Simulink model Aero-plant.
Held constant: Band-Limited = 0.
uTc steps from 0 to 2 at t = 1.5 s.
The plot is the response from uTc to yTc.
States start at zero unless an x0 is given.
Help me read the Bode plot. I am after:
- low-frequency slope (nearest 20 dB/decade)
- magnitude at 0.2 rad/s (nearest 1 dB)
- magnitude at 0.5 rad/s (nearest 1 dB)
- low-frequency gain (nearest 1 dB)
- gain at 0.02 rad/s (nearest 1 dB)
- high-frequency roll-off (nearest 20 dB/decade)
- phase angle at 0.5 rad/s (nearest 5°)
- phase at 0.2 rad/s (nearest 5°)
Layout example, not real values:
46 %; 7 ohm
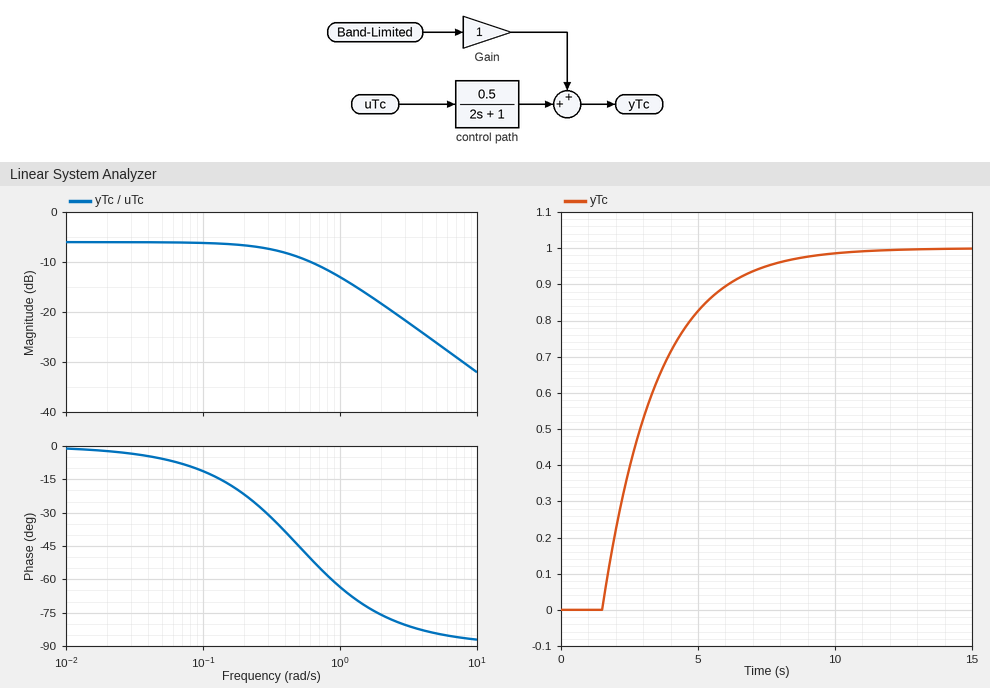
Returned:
0 dB/decade; -7 dB; -9 dB; -6 dB; -6 dB; -20 dB/decade; -45°; -20°
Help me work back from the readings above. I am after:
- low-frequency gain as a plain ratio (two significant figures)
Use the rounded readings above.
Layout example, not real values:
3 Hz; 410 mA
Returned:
0.50
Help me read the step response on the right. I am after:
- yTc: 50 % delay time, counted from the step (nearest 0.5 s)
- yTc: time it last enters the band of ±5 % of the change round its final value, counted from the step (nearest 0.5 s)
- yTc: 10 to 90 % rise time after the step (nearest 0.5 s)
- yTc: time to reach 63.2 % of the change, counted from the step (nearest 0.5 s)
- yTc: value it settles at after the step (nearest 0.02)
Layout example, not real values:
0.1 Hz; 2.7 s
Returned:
1.5 s; 6.0 s; 4.5 s; 2.0 s; 1.00
